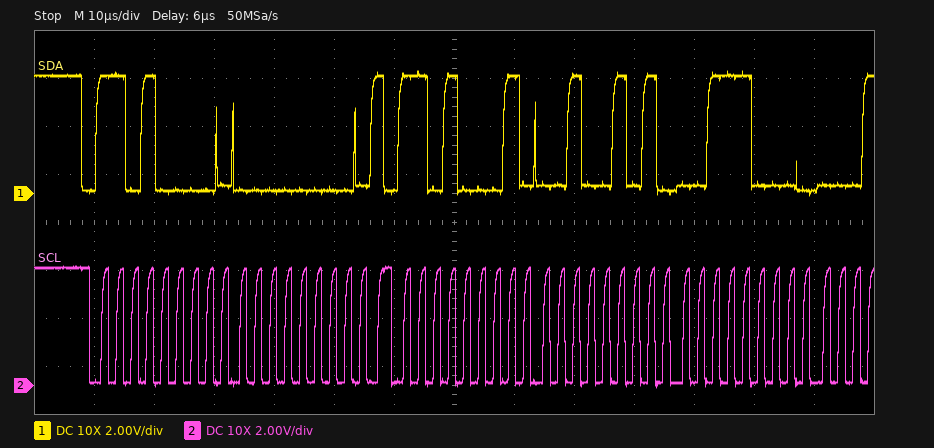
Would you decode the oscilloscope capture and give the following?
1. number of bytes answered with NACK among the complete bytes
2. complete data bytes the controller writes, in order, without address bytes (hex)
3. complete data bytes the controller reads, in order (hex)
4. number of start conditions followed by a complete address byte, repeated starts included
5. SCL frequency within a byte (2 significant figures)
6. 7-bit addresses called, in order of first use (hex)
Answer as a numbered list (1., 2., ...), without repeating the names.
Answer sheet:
1. 0
2. 00
3. 25 38
4. 2
5. 400 kHz
6. 0x68
